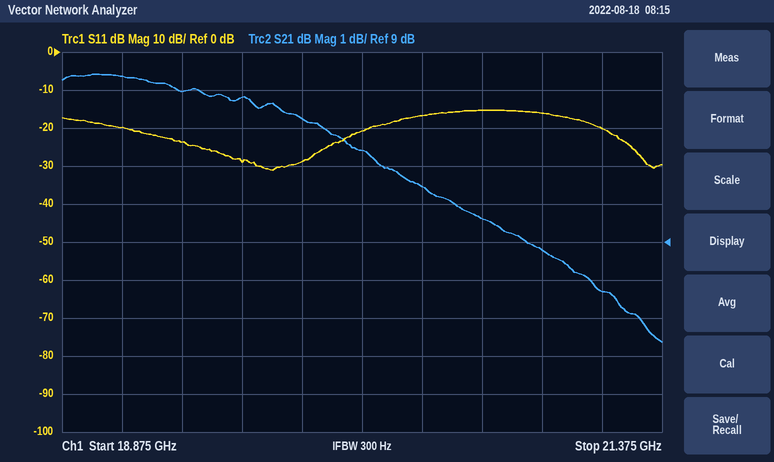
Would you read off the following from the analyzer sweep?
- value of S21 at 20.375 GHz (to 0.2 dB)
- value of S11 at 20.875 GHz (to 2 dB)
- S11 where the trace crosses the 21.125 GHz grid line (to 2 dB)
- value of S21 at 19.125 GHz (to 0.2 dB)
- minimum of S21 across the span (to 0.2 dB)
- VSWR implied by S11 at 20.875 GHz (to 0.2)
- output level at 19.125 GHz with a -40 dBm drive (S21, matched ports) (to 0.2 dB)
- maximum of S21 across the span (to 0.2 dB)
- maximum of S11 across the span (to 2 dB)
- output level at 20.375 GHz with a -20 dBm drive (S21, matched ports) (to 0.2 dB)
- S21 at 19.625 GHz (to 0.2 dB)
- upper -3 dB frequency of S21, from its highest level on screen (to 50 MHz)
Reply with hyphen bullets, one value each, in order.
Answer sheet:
- 10.4 dB
- -16 dB
- -20 dB
- 13.4 dB
- 6.4 dB
- 1.4
- -26.6 dBm
- 13.4 dB
- -16 dB
- -9.6 dBm
- 12.8 dB
- 20.40 GHz
